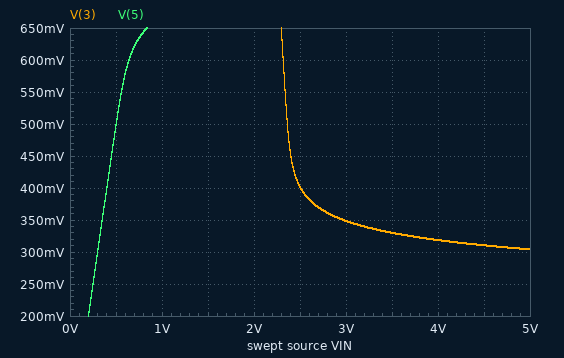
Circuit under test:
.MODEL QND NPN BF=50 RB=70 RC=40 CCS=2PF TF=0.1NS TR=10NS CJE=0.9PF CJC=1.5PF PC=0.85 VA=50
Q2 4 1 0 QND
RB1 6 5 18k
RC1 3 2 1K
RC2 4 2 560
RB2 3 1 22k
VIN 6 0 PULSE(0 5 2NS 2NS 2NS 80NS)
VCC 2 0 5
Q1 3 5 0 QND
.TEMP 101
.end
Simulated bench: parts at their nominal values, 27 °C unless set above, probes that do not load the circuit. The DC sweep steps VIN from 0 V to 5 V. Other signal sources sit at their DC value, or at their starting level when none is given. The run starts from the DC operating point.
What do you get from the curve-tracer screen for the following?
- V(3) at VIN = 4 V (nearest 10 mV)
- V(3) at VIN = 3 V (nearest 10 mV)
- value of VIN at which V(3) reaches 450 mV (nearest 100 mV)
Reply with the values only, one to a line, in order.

320 mV
350 mV
2.4 V
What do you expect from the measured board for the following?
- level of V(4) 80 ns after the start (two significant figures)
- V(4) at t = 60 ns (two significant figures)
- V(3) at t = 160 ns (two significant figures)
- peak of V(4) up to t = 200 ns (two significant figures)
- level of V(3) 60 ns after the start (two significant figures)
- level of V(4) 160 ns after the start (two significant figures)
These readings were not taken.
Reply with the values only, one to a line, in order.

4.1 V
3.1 V
4.3 V
4.6 V
310 mV
2.4 V
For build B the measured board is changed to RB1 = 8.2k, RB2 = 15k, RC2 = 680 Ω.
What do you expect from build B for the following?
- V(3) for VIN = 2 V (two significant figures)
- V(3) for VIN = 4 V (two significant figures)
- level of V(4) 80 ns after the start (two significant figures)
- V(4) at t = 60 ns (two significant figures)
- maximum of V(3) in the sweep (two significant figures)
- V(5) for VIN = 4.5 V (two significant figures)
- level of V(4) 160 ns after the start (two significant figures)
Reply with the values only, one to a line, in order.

330 mV
280 mV
4.3 V
3.4 V
4.7 V
760 mV
560 mV
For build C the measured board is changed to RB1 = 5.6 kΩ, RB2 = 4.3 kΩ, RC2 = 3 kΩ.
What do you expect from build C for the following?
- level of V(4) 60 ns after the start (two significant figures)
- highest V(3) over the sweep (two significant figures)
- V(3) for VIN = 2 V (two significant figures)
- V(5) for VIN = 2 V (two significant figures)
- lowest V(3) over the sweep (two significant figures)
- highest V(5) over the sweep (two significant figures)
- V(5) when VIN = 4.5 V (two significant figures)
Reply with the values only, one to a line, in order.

2.5 V
4.2 V
310 mV
740 mV
260 mV
780 mV
770 mV
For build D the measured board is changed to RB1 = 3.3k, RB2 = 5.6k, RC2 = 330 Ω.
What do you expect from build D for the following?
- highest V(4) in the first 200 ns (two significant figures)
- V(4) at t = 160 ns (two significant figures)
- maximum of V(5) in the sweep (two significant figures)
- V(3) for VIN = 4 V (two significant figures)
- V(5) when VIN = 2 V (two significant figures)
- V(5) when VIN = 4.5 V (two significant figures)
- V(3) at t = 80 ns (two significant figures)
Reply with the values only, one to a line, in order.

5.0 V
650 mV
820 mV
260 mV
750 mV
810 mV
250 mV
